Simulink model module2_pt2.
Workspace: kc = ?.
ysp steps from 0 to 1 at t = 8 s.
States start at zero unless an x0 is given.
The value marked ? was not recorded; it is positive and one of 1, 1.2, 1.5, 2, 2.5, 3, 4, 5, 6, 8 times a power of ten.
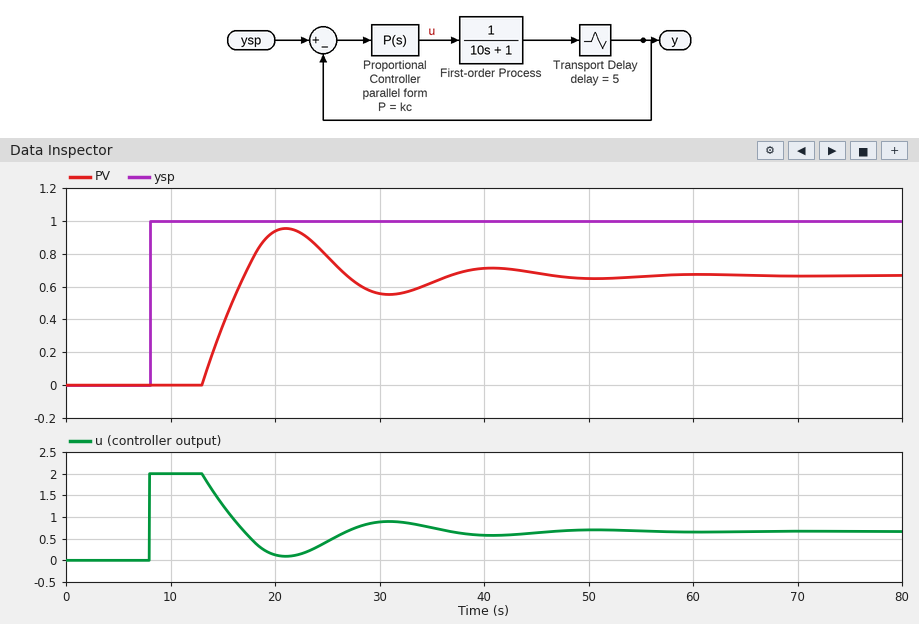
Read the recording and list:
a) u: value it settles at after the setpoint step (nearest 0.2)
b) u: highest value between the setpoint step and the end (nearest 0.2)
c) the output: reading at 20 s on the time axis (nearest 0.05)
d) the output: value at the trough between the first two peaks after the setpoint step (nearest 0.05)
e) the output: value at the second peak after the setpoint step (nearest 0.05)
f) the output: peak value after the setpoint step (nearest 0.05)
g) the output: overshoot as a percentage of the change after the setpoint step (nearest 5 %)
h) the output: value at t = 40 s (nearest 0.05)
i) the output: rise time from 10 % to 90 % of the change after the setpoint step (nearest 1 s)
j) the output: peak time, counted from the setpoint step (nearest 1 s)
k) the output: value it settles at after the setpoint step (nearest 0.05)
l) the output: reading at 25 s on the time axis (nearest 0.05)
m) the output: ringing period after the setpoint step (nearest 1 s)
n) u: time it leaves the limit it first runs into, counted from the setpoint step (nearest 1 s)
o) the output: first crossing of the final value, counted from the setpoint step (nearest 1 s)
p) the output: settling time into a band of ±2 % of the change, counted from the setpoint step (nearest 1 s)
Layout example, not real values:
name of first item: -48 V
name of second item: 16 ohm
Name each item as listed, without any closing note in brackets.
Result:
u: value it settles at after the setpoint step: 0.6
u: highest value between the setpoint step and the end: 2.0
the output: reading at 20 s on the time axis: 0.95
the output: value at the trough between the first two peaks after the setpoint step: 0.55
the output: value at the second peak after the setpoint step: 0.70
the output: peak value after the setpoint step: 0.95
the output: overshoot as a percentage of the change after the setpoint step: 45 %
the output: value at t = 40 s: 0.70
the output: rise time from 10 % to 90 % of the change after the setpoint step: 3 s
the output: peak time, counted from the setpoint step: 13 s
the output: value it settles at after the setpoint step: 0.65
the output: reading at 25 s on the time axis: 0.80
the output: ringing period after the setpoint step: 20 s
u: time it leaves the limit it first runs into, counted from the setpoint step: 5 s
the output: first crossing of the final value, counted from the setpoint step: 9 s
the output: settling time into a band of ±2 % of the change, counted from the setpoint step: 45 s
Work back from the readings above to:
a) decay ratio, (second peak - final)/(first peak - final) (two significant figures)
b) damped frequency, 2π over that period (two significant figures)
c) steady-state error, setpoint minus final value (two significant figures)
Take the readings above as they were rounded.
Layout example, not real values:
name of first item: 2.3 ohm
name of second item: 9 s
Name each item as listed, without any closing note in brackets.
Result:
decay ratio, (second peak - final)/(first peak - final): 0.17
damped frequency, 2π over that period: 0.31 rad/s
steady-state error, setpoint minus final value: 0.35
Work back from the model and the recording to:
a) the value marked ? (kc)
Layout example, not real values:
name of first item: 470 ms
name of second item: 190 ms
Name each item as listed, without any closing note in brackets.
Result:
the value marked ?: 2
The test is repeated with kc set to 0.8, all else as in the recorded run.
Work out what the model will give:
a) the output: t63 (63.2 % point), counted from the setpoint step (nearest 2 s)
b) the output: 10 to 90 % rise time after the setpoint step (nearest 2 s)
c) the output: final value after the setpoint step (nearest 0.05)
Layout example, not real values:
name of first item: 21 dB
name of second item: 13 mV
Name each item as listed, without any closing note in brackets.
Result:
the output: t63 (63.2 % point), counted from the setpoint step: 10 s
the output: 10 to 90 % rise time after the setpoint step: 6 s
the output: final value after the setpoint step: 0.45
